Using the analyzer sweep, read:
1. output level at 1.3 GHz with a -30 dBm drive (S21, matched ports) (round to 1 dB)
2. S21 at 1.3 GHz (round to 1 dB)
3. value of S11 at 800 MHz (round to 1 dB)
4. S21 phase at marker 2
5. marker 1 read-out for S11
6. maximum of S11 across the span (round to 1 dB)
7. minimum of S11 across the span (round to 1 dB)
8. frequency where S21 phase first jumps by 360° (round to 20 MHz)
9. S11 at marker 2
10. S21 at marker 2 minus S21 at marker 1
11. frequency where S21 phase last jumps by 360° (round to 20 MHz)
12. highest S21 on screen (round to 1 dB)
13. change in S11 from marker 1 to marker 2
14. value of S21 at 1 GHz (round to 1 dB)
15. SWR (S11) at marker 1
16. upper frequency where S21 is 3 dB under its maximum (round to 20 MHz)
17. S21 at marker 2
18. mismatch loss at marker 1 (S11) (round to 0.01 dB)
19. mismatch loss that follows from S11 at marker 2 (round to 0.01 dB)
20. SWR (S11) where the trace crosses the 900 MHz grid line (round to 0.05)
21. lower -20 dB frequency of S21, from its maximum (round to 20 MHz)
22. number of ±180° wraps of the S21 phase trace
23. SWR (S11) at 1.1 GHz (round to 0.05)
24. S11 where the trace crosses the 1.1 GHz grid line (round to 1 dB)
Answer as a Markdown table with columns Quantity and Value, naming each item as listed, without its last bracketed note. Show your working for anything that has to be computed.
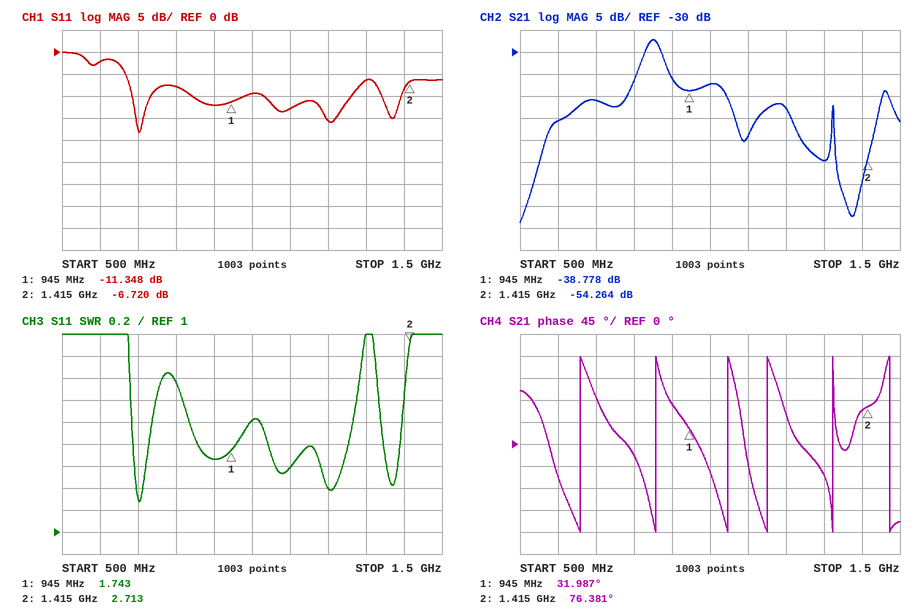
| Quantity | Value |
|---|---|
| output level at 1.3 GHz with a -30 dBm drive (S21, matched ports) | -30 dBm + (-55 dB) = -85 dBm |
| S21 at 1.3 GHz | -55 dB |
| value of S11 at 800 MHz | -8 dB |
| S21 phase at marker 2 | 76.381° |
| marker 1 read-out for S11 | -11.348 dB |
| maximum of S11 across the span | 0 dB |
| minimum of S11 across the span | -18 dB |
| frequency where S21 phase first jumps by 360° | 660 MHz |
| S11 at marker 2 | -6.720 dB |
| S21 at marker 2 minus S21 at marker 1 | -54.264 − (-38.778) = -15.486 dB |
| frequency where S21 phase last jumps by 360° | 1.48 GHz |
| highest S21 on screen | -27 dB |
| change in S11 from marker 1 to marker 2 | -6.72 − (-11.348) = 4.628 dB |
| value of S21 at 1 GHz | -37 dB |
| SWR (S11) at marker 1 | 1.743 |
| upper frequency where S21 is 3 dB under its maximum | 880 MHz |
| S21 at marker 2 | -54.264 dB |
| mismatch loss at marker 1 (S11) | −10 log10(1 − 10^(-11.348/10)) ≈ 0.33 dB |
| mismatch loss that follows from S11 at marker 2 | −10 log10(1 − 10^(-6.72/10)) ≈ 1.04 dB |
| SWR (S11) where the trace crosses the 900 MHz grid line | 1.65 |
| lower -20 dB frequency of S21, from its maximum | 580 MHz |
| number of ±180° wraps of the S21 phase trace | 6 |
| SWR (S11) at 1.1 GHz | 1.60 |
| S11 where the trace crosses the 1.1 GHz grid line | -13 dB |
